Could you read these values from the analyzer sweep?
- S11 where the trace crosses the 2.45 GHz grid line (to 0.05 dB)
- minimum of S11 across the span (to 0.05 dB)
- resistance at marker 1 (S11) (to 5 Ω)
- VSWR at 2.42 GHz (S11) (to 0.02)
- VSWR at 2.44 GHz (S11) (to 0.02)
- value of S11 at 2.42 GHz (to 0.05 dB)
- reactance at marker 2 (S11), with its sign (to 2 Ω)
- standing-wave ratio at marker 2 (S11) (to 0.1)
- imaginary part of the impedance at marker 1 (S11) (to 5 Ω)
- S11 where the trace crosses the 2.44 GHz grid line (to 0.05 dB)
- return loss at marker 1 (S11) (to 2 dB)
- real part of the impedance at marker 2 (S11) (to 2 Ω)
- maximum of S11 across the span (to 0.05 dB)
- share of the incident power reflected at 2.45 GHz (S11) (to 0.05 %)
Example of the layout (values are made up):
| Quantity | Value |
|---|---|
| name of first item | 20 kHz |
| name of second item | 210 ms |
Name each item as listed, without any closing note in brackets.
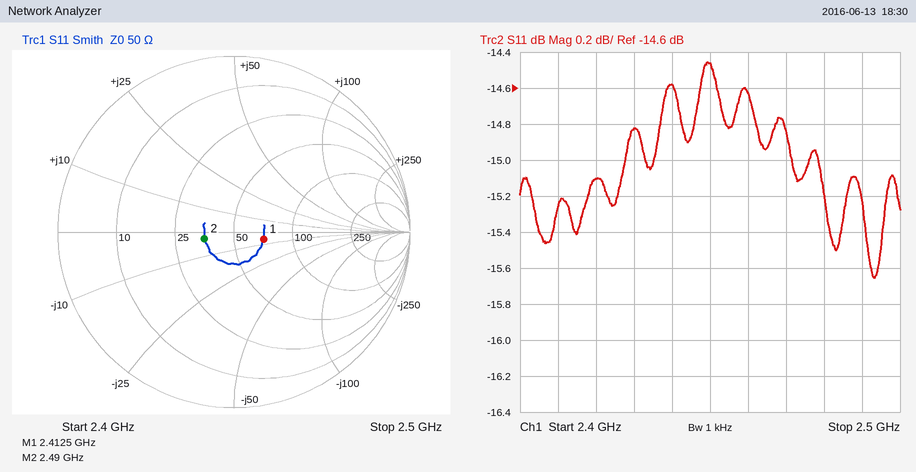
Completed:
| Quantity | Value |
|---|---|
| S11 where the trace crosses the 2.45 GHz grid line | -14.45 dB |
| minimum of S11 across the span | -15.65 dB |
| resistance at marker 1 (S11) | 70 Ω |
| VSWR at 2.42 GHz (S11) | 1.42 |
| VSWR at 2.44 GHz (S11) | 1.46 |
| value of S11 at 2.42 GHz | -15.10 dB |
| reactance at marker 2 (S11), with its sign | -2 Ω |
| standing-wave ratio at marker 2 (S11) | 1.4 |
| imaginary part of the impedance at marker 1 (S11) | -5 Ω |
| S11 where the trace crosses the 2.44 GHz grid line | -14.60 dB |
| return loss at marker 1 (S11) | 16 dB |
| real part of the impedance at marker 2 (S11) | 36 Ω |
| maximum of S11 across the span | -14.45 dB |
| share of the incident power reflected at 2.45 GHz (S11) | 3.60 % |
